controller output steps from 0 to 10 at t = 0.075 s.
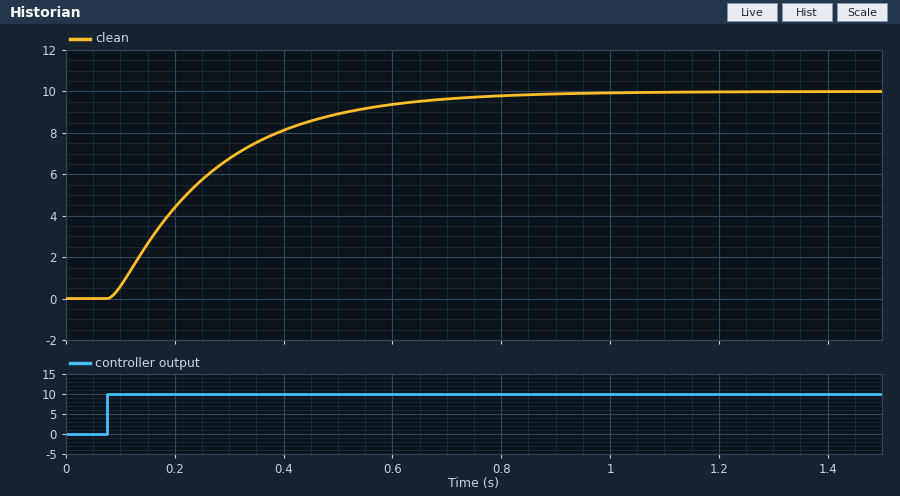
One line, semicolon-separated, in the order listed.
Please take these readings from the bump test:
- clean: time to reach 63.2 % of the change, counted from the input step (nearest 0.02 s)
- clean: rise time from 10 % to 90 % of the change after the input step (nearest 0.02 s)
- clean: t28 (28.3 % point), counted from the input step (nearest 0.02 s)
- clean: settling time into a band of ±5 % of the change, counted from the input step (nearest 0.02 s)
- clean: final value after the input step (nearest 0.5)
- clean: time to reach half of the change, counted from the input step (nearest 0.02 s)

0.20 s; 0.40 s; 0.08 s; 0.56 s; 10.0; 0.14 s
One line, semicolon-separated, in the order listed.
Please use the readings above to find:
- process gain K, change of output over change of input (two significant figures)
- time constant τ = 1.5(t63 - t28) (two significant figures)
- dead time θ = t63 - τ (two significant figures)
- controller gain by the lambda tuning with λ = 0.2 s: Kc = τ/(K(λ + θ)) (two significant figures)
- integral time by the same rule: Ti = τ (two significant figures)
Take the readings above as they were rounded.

1.0; 0.18 s; 0.020 s; 0.82; 0.18 s
